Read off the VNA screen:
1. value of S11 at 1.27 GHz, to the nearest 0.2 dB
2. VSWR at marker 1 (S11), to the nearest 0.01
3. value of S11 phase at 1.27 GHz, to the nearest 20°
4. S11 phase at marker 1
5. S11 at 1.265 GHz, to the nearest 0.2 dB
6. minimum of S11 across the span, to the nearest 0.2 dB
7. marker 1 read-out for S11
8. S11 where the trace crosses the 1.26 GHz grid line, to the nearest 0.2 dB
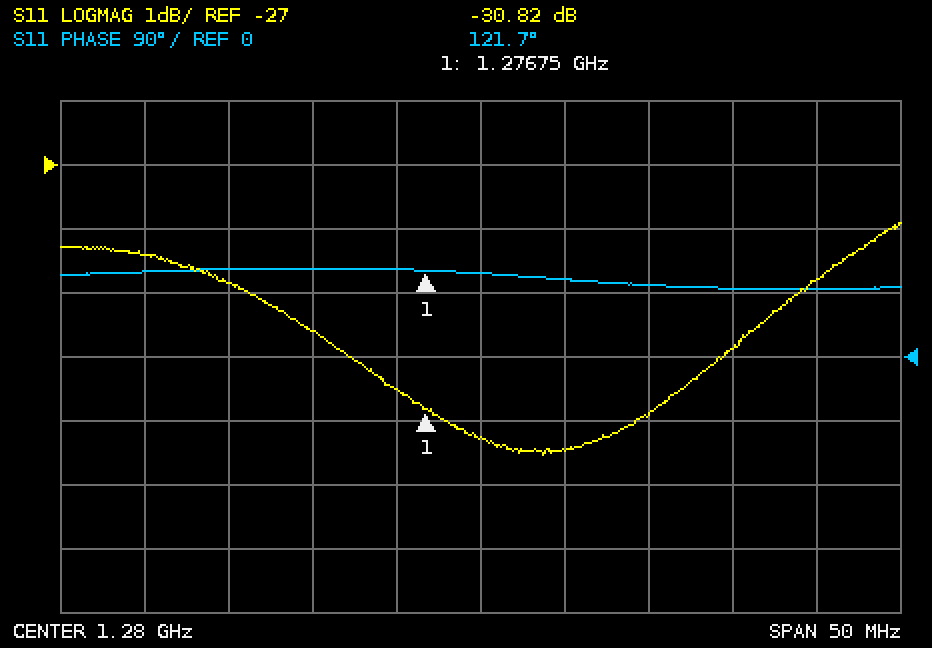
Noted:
-29.6 dB
1.06
120°
121.7°
-28.8 dB
-31.6 dB
-30.82 dB
-28.4 dB
